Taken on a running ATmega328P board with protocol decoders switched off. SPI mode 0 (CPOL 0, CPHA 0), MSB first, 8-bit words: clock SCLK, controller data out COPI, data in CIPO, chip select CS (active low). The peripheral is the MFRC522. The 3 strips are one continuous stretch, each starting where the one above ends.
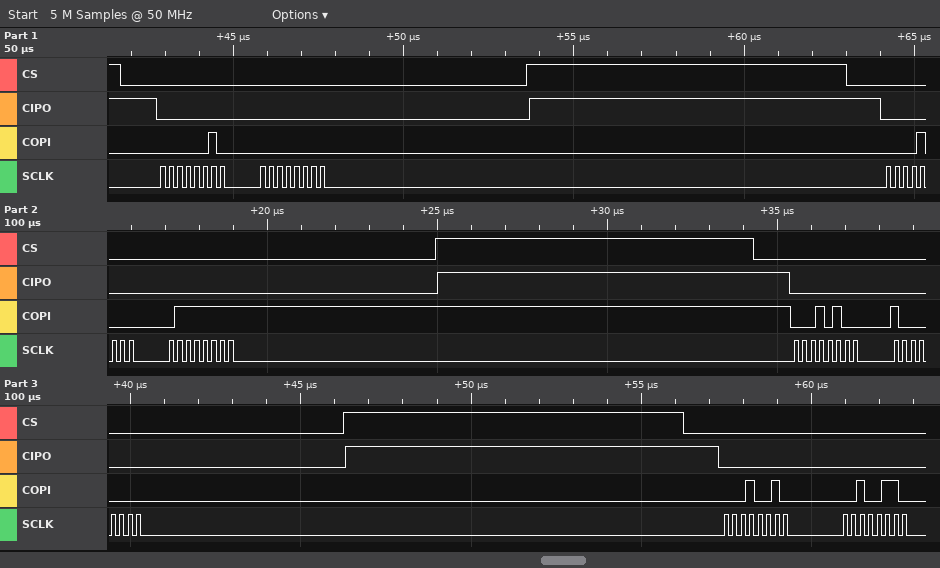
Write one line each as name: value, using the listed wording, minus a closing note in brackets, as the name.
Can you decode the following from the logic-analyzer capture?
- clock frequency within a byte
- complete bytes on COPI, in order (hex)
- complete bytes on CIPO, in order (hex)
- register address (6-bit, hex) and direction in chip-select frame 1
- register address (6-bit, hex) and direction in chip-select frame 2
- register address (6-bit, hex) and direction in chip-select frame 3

clock frequency within a byte: 4 MHz
complete bytes on COPI, in order: 02 00 08 7F 14 80 12 26
complete bytes on CIPO, in order: 00 00 00 00 00 00 00 00
register address (6-bit, hex) and direction in chip-select frame 1: 0x01 write
register address (6-bit, hex) and direction in chip-select frame 2: 0x04 write
register address (6-bit, hex) and direction in chip-select frame 3: 0x0A write
